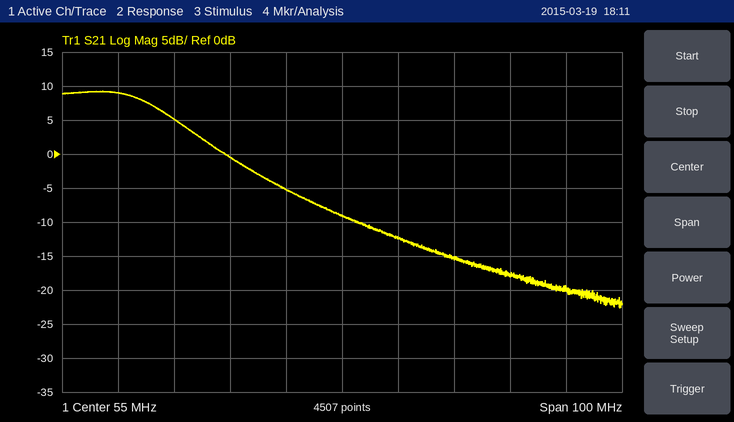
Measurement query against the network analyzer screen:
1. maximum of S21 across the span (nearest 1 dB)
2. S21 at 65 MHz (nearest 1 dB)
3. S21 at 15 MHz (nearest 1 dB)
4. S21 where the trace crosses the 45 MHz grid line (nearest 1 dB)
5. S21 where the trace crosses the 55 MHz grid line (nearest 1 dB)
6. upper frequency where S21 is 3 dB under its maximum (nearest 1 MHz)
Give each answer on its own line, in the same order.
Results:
9 dB
-12 dB
9 dB
-5 dB
-9 dB
23 MHz
